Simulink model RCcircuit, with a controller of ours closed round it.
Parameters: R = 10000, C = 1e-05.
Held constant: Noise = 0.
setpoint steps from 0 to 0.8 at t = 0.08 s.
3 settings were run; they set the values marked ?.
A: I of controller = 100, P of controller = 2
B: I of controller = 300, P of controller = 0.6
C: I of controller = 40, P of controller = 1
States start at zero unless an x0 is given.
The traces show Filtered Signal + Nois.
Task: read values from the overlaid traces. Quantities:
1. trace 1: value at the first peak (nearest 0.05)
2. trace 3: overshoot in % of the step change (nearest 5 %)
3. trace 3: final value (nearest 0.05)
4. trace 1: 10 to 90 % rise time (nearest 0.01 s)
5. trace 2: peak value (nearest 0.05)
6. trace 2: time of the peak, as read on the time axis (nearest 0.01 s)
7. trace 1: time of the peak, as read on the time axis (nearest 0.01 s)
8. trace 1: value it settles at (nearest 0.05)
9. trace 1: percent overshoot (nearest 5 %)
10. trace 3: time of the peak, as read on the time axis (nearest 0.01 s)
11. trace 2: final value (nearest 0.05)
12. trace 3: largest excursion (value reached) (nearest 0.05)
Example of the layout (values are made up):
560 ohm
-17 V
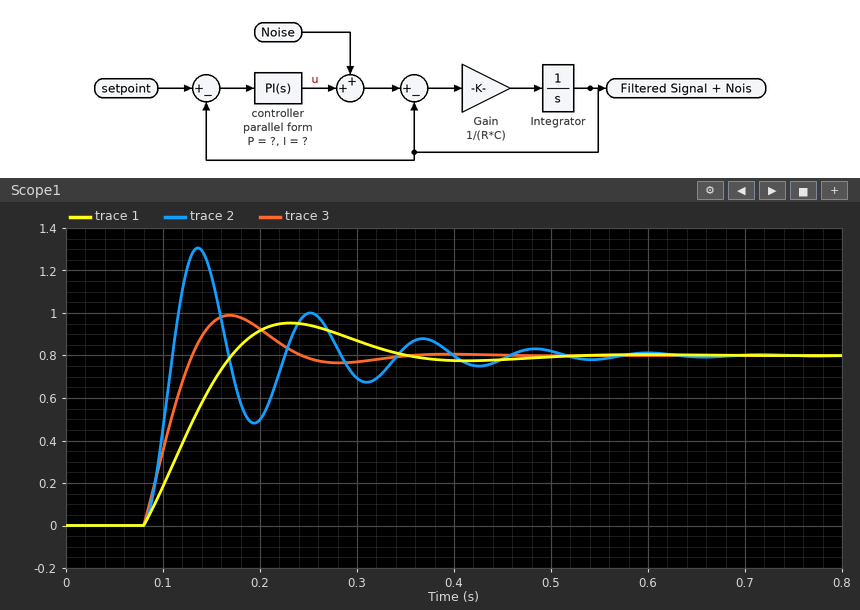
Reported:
0.95
25 %
0.80
0.07 s
1.30
0.14 s
0.23 s
0.80
20 %
0.17 s
0.80
1.00
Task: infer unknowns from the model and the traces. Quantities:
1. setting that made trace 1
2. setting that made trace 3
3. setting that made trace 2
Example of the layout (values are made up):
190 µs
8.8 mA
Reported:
C
A
B
